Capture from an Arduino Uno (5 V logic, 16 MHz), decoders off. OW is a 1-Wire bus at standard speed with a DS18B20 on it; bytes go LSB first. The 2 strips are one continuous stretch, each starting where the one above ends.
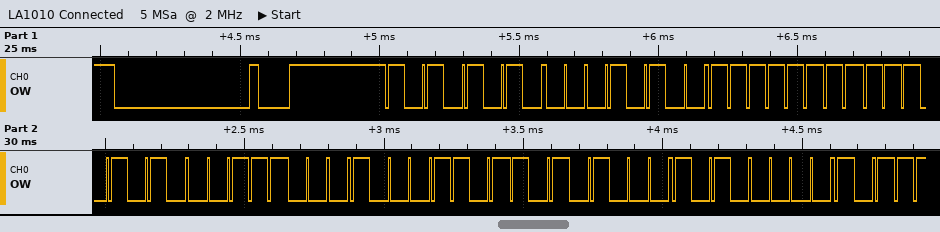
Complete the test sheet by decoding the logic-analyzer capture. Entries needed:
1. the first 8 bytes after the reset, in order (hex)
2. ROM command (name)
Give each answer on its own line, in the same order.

55 28 FF 57 1C B1 15 05
Match ROM
